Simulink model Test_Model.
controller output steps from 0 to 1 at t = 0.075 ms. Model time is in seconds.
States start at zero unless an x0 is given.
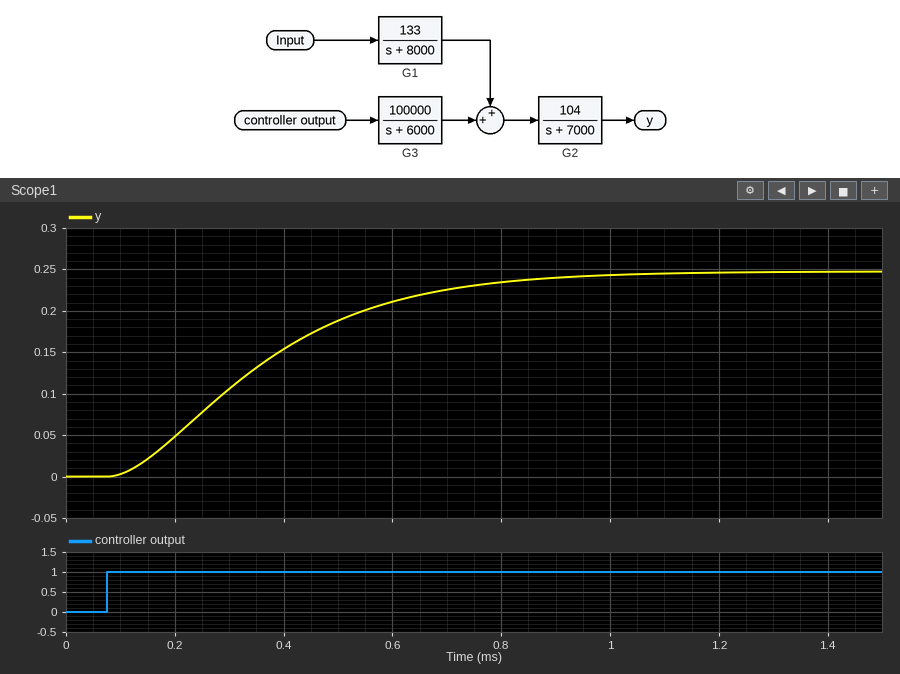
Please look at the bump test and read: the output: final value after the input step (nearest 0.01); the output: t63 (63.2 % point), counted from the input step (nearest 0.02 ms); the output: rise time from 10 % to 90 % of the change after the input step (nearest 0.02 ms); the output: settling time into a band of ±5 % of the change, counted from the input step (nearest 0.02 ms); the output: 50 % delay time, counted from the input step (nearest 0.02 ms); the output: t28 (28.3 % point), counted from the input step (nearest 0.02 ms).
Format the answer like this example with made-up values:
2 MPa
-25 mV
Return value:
0.25
0.34 ms
0.52 ms
0.74 ms
0.26 ms
0.16 ms
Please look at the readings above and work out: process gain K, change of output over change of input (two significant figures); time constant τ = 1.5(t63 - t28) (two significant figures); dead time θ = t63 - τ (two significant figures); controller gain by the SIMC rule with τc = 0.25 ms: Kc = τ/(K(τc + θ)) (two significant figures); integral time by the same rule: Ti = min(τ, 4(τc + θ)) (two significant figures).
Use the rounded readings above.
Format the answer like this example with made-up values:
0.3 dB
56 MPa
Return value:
0.25
0.27 ms
0.070 ms
3.4
0.27 ms
